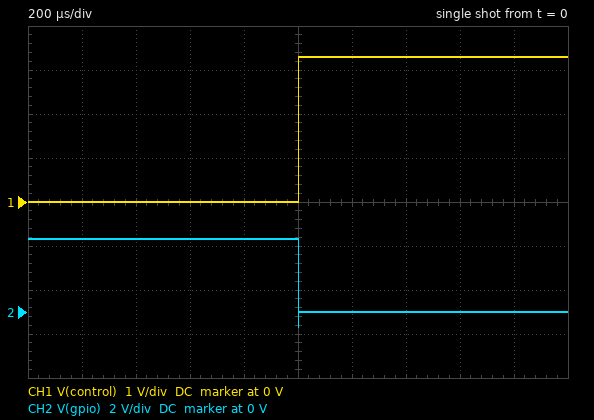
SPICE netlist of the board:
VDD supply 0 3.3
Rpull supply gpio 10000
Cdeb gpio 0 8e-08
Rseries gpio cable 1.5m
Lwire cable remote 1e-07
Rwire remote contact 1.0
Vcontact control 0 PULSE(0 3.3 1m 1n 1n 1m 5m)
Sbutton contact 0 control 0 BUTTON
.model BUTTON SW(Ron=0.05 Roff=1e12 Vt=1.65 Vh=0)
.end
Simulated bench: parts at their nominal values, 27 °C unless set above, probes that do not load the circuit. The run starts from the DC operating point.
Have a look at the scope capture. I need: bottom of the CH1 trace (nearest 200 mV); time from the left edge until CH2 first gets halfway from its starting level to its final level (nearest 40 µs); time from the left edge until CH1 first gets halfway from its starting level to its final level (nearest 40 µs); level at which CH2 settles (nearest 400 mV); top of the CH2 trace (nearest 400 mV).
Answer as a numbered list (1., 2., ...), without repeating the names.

1. 0 V
2. 1.00 ms
3. 1.00 ms
4. 0 V
5. 3.2 V
